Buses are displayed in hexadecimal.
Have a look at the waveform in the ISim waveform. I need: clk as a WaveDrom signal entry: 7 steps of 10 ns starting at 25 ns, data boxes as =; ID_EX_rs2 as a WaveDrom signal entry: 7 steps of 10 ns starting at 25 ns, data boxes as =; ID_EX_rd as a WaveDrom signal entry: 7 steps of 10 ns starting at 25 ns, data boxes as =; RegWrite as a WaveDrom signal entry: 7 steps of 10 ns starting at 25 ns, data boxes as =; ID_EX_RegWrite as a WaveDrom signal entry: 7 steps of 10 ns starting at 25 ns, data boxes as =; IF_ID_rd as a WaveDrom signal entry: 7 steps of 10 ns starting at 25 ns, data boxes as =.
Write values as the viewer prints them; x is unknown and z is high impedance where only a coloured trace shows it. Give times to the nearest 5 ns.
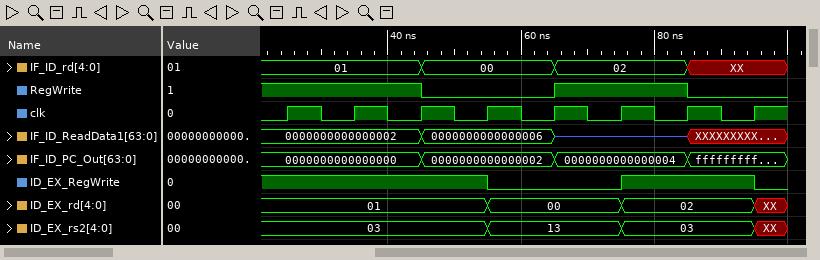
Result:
{name: 'clk', wave: 'p......'}
{name: 'ID_EX_rs2', wave: '=..=.=.', data: '03 13 03'}
{name: 'ID_EX_rd', wave: '=..=.=.', data: '01 00 02'}
{name: 'RegWrite', wave: '1.0.1.0'}
{name: 'ID_EX_RegWrite', wave: '1..0.1.'}
{name: 'IF_ID_rd', wave: '=.=.=.x', data: '01 00 02'}
